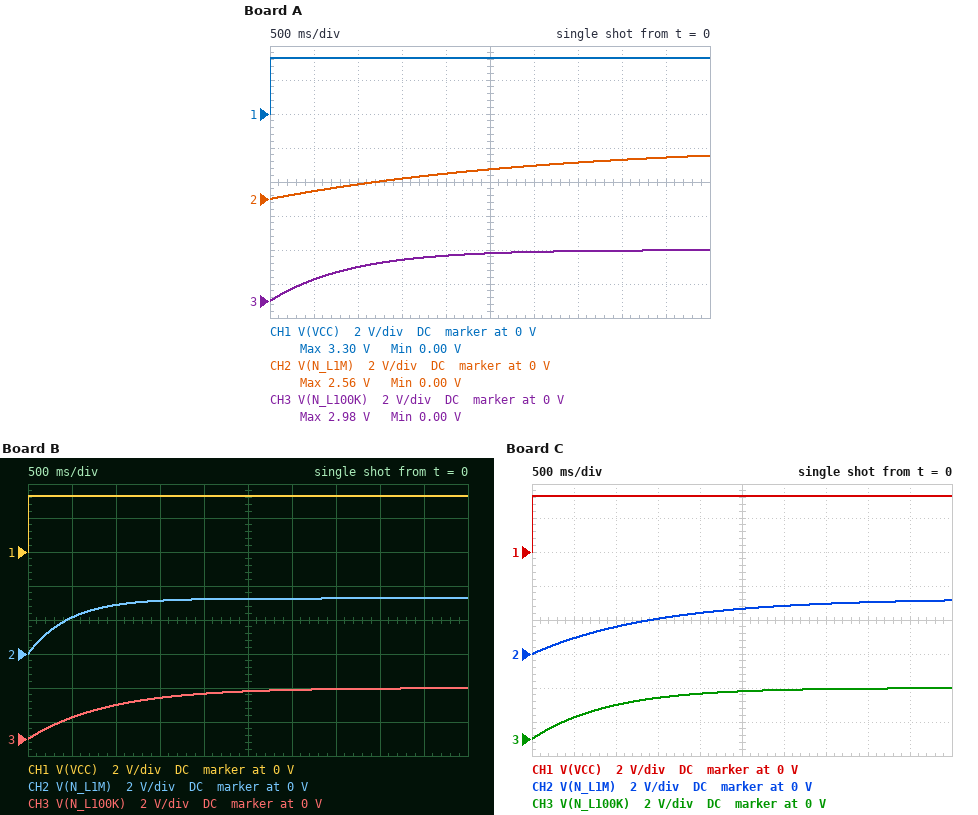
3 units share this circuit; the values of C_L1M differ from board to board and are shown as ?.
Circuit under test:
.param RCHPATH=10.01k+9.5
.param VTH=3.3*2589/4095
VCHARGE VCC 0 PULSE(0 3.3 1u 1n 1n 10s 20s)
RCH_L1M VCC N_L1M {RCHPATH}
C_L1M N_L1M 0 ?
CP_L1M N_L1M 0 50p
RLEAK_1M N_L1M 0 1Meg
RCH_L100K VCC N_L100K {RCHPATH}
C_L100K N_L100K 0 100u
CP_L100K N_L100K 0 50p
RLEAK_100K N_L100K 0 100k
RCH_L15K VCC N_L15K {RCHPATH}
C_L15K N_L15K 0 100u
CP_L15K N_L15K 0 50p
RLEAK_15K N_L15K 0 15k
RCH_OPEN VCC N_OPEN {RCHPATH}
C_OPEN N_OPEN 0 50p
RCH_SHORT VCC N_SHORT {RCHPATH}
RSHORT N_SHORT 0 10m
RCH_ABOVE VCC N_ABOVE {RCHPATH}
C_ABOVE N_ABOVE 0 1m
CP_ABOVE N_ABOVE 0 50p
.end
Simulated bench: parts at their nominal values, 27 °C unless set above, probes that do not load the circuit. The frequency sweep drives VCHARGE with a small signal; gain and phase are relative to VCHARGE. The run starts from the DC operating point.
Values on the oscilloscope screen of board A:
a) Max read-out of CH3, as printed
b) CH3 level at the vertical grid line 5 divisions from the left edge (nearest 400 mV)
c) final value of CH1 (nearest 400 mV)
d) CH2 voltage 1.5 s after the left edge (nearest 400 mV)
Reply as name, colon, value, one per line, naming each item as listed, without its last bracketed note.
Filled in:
Max read-out of CH3, as printed: 2.98 V
CH3 level at the vertical grid line 5 divisions from the left edge: 2.8 V
final value of CH1: 3.2 V
CH2 voltage 1.5 s after the left edge: 1.2 V
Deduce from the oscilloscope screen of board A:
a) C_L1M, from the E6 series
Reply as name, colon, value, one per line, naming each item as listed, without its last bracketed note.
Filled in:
C_L1M, from the E6 series: 330 µF
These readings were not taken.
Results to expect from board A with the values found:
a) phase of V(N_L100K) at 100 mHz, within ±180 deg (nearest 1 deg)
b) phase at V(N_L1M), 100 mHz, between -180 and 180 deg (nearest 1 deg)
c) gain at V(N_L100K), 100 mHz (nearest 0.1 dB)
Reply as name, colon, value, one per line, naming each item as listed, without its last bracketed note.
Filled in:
phase of V(N_L100K) at 100 mHz, within ±180 deg: -30 deg
phase at V(N_L1M), 100 mHz, between -180 and 180 deg: -64 deg
gain at V(N_L100K), 100 mHz: -2.1 dB
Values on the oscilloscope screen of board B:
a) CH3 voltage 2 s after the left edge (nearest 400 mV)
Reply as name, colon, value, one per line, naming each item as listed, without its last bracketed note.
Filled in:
CH3 voltage 2 s after the left edge: 2.8 V
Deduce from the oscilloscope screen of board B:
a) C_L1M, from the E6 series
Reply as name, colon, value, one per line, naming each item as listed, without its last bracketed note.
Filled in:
C_L1M, from the E6 series: 47 µF
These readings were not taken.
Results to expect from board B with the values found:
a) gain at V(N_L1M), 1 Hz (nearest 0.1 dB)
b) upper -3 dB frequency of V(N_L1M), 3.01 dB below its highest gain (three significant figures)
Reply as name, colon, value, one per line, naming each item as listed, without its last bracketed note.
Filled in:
gain at V(N_L1M), 1 Hz: -9.9 dB
upper -3 dB frequency of V(N_L1M), 3.01 dB below its highest gain: 341 mHz
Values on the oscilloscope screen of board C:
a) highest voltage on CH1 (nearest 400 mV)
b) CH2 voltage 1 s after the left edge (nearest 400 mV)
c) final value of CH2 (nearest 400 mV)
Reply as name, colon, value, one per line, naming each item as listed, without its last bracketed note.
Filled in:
highest voltage on CH1: 3.2 V
CH2 voltage 1 s after the left edge: 1.6 V
final value of CH2: 3.2 V
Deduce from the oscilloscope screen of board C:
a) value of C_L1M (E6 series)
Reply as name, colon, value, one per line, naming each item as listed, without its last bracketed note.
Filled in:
value of C_L1M: 150 µF
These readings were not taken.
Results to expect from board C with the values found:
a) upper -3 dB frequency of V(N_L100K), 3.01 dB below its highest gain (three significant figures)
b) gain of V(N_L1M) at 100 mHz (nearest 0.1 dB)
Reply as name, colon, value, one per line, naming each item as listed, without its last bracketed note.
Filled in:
upper -3 dB frequency of V(N_L100K), 3.01 dB below its highest gain: 175 mHz
gain of V(N_L1M) at 100 mHz: -2.8 dB
